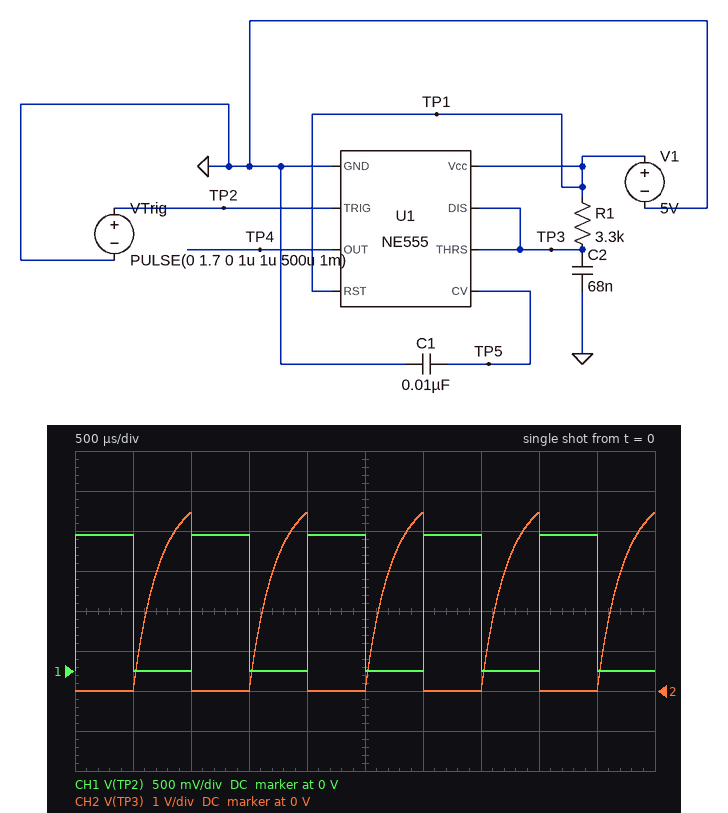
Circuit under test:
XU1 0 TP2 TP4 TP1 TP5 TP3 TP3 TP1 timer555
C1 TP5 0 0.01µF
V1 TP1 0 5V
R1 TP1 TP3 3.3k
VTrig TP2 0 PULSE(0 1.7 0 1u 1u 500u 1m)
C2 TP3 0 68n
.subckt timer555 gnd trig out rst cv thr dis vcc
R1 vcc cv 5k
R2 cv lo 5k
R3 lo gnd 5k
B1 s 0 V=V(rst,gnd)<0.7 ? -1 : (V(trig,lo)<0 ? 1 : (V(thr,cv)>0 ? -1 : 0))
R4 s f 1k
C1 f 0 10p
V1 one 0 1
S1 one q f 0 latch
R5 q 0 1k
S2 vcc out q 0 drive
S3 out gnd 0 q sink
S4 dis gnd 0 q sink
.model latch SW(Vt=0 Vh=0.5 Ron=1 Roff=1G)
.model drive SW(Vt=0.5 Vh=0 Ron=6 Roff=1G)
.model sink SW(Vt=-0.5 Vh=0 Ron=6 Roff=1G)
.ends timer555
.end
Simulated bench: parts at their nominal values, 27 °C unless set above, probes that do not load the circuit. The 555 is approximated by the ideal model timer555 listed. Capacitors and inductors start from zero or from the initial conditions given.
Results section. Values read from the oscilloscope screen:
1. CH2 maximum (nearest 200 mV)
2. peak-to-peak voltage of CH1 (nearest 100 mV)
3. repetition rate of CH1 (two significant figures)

4.4 V
1.7 V
1.0 kHz
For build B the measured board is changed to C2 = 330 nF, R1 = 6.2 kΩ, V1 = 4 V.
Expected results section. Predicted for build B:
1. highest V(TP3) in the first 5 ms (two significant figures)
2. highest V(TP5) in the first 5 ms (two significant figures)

2.8 V
2.7 V
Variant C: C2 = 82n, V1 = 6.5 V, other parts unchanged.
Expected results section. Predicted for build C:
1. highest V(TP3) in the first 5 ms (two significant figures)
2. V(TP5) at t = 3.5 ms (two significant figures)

6.5 V
4.3 V
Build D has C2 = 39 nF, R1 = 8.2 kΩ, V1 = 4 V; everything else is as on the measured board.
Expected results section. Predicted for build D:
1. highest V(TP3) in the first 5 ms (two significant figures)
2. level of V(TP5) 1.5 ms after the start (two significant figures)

3.2 V
2.7 V
